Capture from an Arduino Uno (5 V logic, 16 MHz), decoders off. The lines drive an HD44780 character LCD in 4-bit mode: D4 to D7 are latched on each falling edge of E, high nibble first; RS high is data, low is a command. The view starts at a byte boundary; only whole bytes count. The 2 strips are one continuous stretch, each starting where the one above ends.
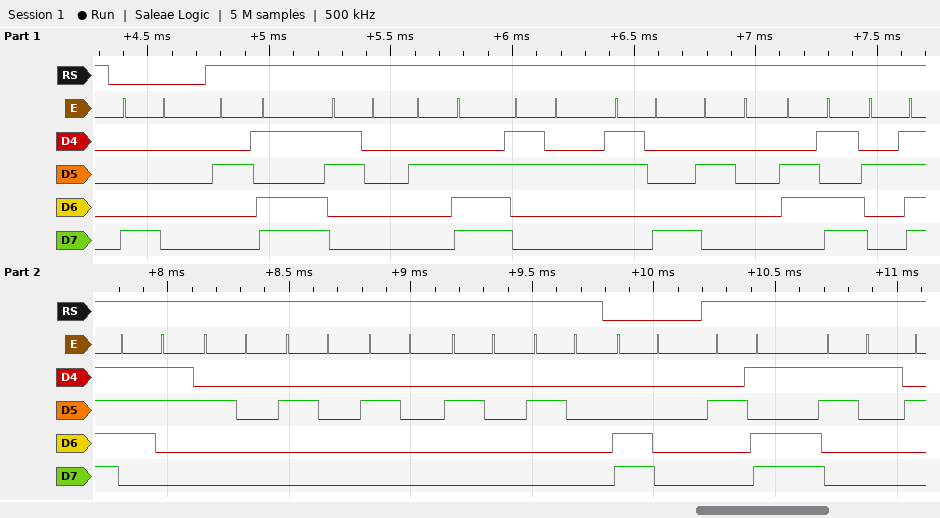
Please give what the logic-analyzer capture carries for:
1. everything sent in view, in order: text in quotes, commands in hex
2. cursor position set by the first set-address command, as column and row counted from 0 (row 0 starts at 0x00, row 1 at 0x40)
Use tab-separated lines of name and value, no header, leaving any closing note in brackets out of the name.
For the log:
everything sent in view, in order: text in quotes, commands in hex	0x80 "-0.28 m/s     " 0xC0 "-1"
cursor position set by the first set-address command, as column and row counted from 0	column 0, row 0
